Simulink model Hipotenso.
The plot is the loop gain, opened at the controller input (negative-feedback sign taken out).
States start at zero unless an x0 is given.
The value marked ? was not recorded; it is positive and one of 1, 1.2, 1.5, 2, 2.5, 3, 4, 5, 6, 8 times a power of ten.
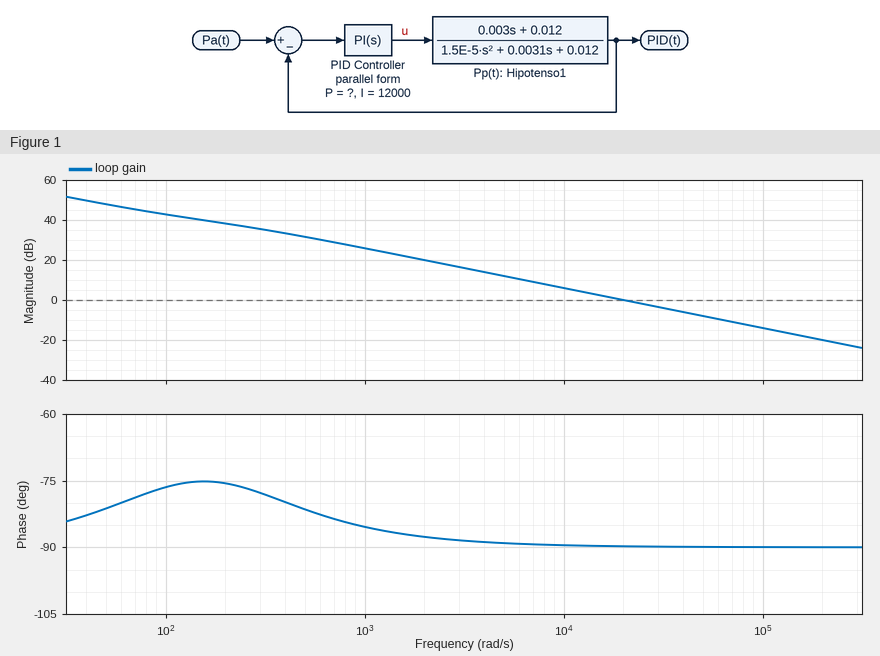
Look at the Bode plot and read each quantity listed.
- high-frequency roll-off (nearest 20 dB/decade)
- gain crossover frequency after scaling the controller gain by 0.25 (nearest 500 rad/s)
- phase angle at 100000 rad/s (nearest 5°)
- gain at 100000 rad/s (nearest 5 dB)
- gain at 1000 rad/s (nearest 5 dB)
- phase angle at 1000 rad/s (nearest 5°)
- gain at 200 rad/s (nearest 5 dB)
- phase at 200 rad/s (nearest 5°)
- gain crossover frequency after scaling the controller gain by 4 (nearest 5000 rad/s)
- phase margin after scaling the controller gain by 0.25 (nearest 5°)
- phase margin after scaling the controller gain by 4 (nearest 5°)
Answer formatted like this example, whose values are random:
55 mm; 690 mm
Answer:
-20 dB/decade; 5000 rad/s; -90°; -15 dB; 25 dB; -85°; 40 dB; -75°; 80000 rad/s; 90°; 90°
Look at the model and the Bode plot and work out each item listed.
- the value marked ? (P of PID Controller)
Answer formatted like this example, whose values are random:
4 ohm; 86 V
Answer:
100
